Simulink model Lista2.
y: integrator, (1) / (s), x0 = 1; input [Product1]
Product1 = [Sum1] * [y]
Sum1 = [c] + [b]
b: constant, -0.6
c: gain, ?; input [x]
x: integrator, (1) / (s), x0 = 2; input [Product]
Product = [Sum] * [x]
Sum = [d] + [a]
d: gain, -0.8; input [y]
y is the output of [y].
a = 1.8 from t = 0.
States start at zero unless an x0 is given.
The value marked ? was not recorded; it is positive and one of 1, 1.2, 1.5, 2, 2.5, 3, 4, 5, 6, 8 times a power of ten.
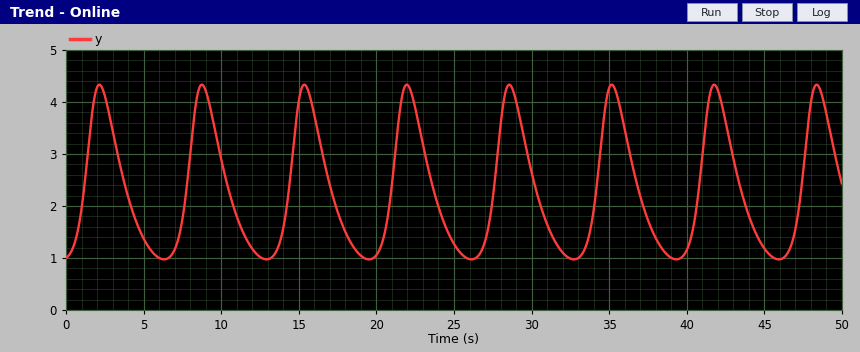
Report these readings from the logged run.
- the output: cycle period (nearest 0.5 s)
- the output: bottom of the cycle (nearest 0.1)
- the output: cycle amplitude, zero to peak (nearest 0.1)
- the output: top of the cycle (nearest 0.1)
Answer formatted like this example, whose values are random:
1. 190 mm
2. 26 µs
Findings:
1. 6.5 s
2. 1.0
3. 1.7
4. 4.3
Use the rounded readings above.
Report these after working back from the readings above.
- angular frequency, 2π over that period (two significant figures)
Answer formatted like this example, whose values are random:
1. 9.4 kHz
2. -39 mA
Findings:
1. 0.97 rad/s
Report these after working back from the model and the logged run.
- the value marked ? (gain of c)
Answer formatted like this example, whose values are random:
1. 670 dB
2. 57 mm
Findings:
1. 0.4
